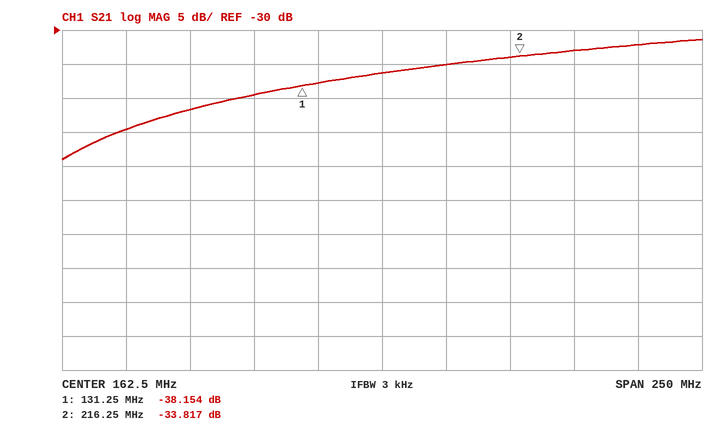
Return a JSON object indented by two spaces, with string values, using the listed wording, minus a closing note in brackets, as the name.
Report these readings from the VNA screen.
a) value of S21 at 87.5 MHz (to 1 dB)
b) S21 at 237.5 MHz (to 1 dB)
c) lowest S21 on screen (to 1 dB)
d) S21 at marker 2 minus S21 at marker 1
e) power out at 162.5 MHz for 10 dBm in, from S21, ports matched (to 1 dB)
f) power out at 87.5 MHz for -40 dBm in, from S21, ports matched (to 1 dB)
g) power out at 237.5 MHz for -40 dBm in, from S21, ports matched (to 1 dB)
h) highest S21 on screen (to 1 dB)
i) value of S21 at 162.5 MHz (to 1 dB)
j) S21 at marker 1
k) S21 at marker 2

{
  "value of S21 at 87.5 MHz": "-42 dB",
  "S21 at 237.5 MHz": "-33 dB",
  "lowest S21 on screen": "-49 dB",
  "S21 at marker 2 minus S21 at marker 1": "4.337 dB",
  "power out at 162.5 MHz for 10 dBm in, from S21, ports matched": "-26 dBm",
  "power out at 87.5 MHz for -40 dBm in, from S21, ports matched": "-82 dBm",
  "power out at 237.5 MHz for -40 dBm in, from S21, ports matched": "-73 dBm",
  "highest S21 on screen": "-31 dB",
  "value of S21 at 162.5 MHz": "-36 dB",
  "S21 at marker 1": "-38.154 dB",
  "S21 at marker 2": "-33.817 dB"
}
